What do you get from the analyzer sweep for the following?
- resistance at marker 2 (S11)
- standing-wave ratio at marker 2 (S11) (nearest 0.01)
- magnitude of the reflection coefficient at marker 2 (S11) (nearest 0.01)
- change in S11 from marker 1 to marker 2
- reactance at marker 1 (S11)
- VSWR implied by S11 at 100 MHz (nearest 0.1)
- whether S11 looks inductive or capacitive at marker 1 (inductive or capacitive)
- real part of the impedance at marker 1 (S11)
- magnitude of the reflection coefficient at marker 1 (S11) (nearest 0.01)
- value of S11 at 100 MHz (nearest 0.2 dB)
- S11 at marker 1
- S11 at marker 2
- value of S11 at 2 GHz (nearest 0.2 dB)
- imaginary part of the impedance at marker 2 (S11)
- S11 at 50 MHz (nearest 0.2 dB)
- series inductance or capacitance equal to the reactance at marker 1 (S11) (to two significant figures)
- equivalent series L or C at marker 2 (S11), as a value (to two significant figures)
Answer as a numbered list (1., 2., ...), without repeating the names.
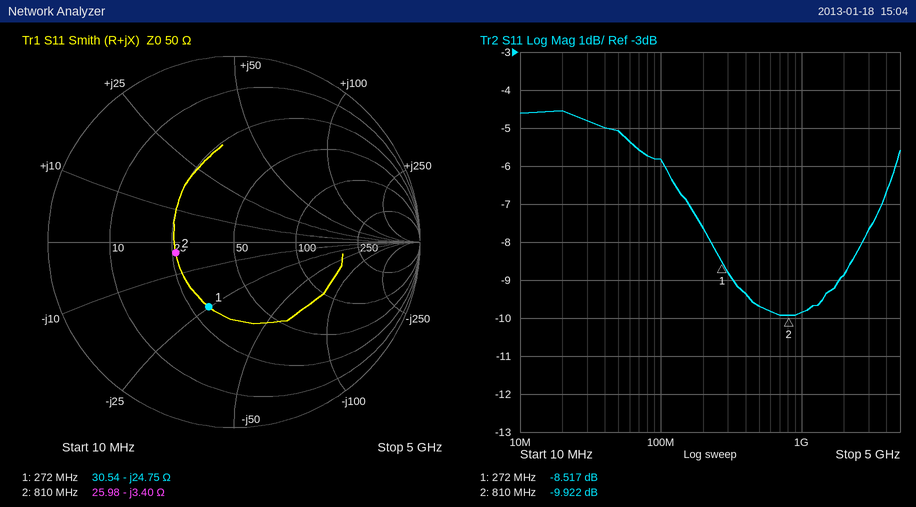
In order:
1. 25.98 Ω
2. 1.94
3. 0.32
4. -1.405 dB
5. -24.75 Ω
6. 3.1
7. capacitive
8. 30.54 Ω
9. 0.37
10. -5.8 dB
11. -8.517 dB
12. -9.922 dB
13. -8.8 dB
14. -3.40 Ω
15. -5.0 dB
16. 24 pF
17. 58 pF
